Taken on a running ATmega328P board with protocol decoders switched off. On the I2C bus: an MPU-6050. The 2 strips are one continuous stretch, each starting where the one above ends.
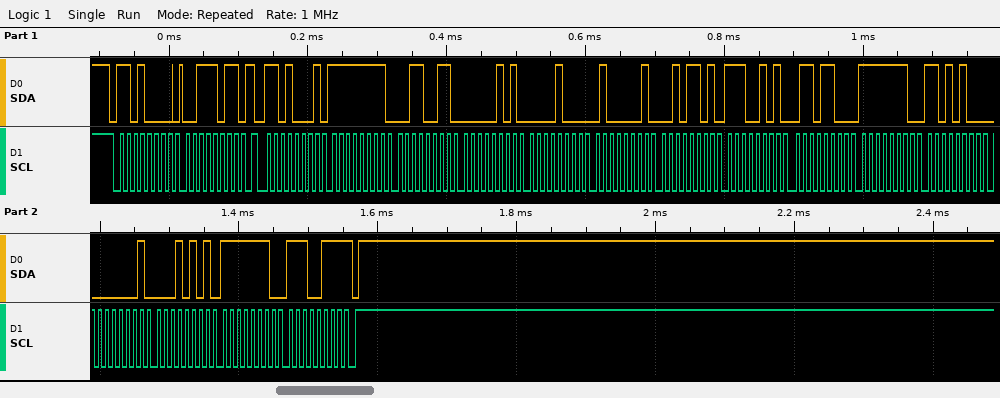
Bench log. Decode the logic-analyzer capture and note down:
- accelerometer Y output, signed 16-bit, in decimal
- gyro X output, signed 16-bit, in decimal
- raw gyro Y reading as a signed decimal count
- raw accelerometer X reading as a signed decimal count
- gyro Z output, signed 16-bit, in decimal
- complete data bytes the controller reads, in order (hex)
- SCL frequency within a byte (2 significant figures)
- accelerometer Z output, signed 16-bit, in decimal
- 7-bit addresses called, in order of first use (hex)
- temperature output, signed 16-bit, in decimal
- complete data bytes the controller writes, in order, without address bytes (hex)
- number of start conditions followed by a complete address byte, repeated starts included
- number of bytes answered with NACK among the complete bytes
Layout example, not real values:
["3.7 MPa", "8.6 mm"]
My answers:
["1288", "-300", "277", "-205", "-281", "FF 33 05 08 41 2D E5 6C FE D4 01 15 FE E7", "100 kHz", "16685", "0x68", "-6804", "3B", "2", "1"]
